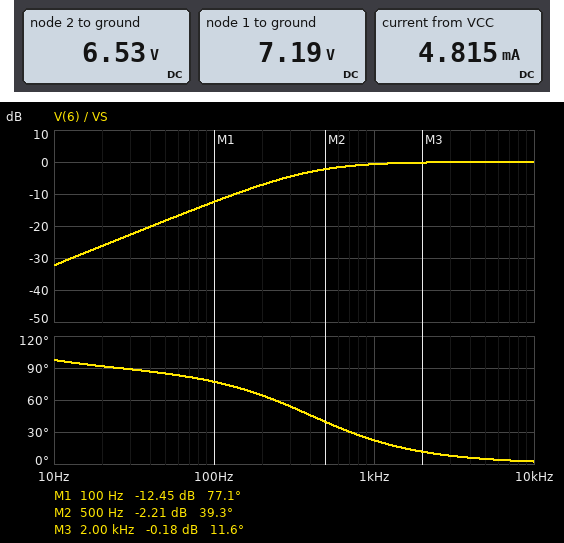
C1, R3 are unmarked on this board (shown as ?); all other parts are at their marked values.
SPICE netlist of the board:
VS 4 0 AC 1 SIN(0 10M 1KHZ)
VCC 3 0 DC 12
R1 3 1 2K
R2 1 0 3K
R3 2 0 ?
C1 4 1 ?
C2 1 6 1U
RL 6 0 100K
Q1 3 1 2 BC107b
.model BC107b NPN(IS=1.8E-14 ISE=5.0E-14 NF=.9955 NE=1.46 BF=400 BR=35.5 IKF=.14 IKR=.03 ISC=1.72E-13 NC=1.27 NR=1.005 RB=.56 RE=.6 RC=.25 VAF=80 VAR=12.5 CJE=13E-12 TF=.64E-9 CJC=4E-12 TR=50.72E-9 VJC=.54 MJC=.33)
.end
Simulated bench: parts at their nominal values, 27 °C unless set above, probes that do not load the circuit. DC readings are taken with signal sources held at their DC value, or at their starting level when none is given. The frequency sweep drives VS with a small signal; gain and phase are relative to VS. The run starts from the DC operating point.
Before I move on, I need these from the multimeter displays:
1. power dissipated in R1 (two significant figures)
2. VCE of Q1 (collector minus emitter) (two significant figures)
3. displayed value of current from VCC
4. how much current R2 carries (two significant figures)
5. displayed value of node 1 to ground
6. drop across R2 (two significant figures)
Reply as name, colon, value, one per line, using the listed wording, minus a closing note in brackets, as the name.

power dissipated in R1: 12 mW
VCE of Q1 (collector minus emitter): 5.5 V
displayed value of current from VCC: 4.815 mA
how much current R2 carries: 2.4 mA
displayed value of node 1 to ground: 7.19 V
drop across R2: 7.2 V
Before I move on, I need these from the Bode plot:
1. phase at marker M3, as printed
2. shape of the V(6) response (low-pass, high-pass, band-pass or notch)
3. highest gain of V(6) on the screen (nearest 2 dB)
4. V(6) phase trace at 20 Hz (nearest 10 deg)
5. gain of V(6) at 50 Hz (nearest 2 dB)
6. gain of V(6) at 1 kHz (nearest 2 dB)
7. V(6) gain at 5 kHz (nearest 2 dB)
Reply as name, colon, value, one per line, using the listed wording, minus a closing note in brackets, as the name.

phase at marker M3, as printed: 11.6 deg
shape of the V(6) response: high-pass
highest gain of V(6) on the screen: 0 dB
V(6) phase trace at 20 Hz: 90 deg
gain of V(6) at 50 Hz: -18 dB
gain of V(6) at 1 kHz: 0 dB
V(6) gain at 5 kHz: 0 dB
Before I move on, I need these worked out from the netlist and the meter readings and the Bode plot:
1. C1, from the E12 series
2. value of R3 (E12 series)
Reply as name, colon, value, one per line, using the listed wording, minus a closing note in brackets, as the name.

C1, from the E12 series: 330 nF
value of R3: 2.7 kΩ
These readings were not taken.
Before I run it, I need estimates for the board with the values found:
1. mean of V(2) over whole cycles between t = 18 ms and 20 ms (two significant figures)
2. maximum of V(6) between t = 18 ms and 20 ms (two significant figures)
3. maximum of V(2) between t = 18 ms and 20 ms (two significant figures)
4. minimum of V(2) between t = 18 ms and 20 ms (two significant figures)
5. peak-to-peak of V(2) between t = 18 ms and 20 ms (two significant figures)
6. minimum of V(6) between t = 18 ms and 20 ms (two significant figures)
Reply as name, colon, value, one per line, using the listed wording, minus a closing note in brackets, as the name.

mean of V(2) over whole cycles between t = 18 ms and 20 ms: 6.5 V
maximum of V(6) between t = 18 ms and 20 ms: 9.3 mV
maximum of V(2) between t = 18 ms and 20 ms: 6.5 V
minimum of V(2) between t = 18 ms and 20 ms: 6.5 V
peak-to-peak of V(2) between t = 18 ms and 20 ms: 18 mV
minimum of V(6) between t = 18 ms and 20 ms: -9.3 mV
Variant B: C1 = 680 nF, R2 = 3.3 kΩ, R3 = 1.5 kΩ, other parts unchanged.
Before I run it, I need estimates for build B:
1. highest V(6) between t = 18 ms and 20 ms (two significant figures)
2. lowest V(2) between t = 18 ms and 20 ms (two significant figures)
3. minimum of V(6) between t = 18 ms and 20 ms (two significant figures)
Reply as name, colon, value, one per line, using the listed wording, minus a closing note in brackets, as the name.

highest V(6) between t = 18 ms and 20 ms: 9.8 mV
lowest V(2) between t = 18 ms and 20 ms: 6.8 V
minimum of V(6) between t = 18 ms and 20 ms: -9.8 mV
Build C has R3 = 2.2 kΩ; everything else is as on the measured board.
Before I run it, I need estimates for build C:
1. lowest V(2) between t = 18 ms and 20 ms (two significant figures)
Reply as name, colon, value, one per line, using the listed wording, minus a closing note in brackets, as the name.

lowest V(2) between t = 18 ms and 20 ms: 6.5 V
